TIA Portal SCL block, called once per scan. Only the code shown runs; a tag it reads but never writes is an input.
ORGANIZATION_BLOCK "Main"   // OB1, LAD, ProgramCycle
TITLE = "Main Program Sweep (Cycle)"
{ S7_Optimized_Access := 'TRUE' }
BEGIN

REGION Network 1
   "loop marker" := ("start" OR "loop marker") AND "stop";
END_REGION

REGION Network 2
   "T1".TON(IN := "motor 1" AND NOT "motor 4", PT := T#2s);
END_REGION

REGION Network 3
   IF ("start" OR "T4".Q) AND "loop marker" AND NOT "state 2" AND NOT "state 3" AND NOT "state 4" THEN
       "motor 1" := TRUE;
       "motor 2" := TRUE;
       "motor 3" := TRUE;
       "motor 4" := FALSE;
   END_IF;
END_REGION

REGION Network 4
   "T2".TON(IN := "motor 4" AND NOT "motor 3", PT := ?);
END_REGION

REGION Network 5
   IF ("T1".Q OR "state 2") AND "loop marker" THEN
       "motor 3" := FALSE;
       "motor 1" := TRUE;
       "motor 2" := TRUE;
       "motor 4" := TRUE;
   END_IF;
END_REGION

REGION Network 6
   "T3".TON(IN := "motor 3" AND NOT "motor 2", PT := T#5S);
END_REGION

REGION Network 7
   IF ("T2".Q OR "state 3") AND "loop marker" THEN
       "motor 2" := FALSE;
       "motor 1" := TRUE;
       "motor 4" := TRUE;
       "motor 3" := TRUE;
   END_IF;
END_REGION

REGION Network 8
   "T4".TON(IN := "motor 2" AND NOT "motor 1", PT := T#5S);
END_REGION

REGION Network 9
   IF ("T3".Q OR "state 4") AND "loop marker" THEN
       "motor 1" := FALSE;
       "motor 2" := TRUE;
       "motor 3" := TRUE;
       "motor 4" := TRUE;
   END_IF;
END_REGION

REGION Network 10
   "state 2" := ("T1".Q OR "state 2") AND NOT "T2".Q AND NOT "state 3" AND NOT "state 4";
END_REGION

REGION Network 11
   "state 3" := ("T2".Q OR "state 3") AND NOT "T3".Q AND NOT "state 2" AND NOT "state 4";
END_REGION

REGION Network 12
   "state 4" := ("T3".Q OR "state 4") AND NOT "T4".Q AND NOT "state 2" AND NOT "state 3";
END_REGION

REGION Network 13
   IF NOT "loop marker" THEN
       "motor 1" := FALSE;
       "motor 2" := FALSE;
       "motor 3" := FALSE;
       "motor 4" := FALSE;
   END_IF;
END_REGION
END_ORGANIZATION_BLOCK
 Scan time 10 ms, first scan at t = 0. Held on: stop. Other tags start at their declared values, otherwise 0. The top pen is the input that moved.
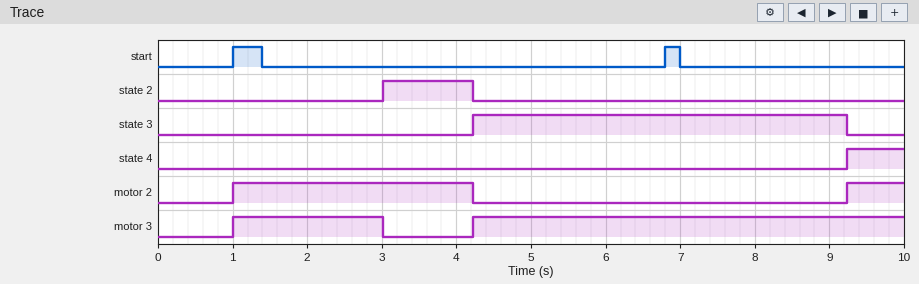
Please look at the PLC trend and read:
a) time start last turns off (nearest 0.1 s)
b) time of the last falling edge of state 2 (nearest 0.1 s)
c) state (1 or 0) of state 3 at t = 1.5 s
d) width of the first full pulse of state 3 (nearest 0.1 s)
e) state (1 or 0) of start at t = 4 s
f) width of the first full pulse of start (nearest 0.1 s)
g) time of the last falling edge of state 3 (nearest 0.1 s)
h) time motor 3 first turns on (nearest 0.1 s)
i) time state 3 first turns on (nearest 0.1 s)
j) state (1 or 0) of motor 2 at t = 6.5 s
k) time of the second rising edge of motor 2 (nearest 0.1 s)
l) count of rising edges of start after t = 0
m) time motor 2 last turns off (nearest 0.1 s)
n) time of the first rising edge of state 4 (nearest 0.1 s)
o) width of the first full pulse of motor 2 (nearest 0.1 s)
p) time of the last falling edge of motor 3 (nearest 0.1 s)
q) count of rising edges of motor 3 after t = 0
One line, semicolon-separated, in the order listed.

7.0 s; 4.2 s; 0; 5.0 s; 0; 0.4 s; 9.2 s; 1.0 s; 4.2 s; 0; 9.2 s; 2; 4.2 s; 9.2 s; 3.2 s; 3.0 s; 2
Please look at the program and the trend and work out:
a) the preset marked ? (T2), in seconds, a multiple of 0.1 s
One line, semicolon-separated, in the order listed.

1.2 s
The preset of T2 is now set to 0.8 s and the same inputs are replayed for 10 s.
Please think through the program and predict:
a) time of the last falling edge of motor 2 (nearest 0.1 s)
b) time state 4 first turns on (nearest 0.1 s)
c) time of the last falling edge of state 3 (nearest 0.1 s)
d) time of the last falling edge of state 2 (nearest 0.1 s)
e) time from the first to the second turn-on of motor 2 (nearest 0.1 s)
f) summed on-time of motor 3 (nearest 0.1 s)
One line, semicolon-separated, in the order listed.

3.8 s; 8.8 s; 8.8 s; 3.8 s; 7.8 s; 8.2 s
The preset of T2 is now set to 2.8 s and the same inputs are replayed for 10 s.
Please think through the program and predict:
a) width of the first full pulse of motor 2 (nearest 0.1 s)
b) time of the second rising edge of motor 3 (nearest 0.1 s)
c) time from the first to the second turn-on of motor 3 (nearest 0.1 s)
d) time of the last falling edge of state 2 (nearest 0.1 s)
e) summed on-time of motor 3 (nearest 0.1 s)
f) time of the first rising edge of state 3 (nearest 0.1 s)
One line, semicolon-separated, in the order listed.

4.8 s; 5.8 s; 4.8 s; 5.8 s; 6.2 s; 5.8 s
